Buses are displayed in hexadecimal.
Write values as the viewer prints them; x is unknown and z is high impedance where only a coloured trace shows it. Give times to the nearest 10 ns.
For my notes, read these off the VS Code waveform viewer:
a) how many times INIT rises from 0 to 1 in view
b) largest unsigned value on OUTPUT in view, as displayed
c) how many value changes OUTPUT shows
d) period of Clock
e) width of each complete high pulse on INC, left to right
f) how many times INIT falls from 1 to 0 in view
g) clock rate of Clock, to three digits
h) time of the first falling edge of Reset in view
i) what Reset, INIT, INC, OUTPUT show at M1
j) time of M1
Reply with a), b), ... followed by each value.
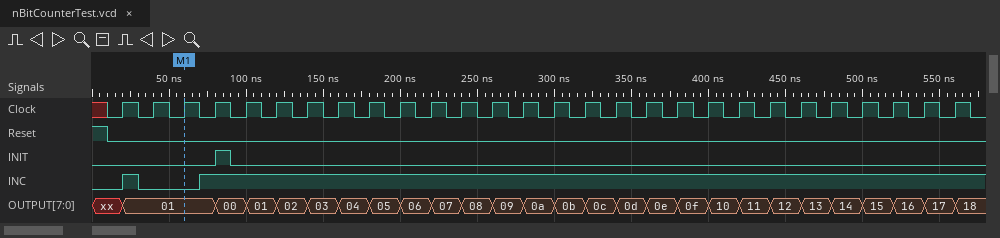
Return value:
a) 1
b) 18
c) 26
d) 20 ns
e) 10 ns
f) 1
g) 50.0 MHz
h) 10 ns
i) Reset=0, INIT=0, INC=0, OUTPUT=01
j) 60 ns
